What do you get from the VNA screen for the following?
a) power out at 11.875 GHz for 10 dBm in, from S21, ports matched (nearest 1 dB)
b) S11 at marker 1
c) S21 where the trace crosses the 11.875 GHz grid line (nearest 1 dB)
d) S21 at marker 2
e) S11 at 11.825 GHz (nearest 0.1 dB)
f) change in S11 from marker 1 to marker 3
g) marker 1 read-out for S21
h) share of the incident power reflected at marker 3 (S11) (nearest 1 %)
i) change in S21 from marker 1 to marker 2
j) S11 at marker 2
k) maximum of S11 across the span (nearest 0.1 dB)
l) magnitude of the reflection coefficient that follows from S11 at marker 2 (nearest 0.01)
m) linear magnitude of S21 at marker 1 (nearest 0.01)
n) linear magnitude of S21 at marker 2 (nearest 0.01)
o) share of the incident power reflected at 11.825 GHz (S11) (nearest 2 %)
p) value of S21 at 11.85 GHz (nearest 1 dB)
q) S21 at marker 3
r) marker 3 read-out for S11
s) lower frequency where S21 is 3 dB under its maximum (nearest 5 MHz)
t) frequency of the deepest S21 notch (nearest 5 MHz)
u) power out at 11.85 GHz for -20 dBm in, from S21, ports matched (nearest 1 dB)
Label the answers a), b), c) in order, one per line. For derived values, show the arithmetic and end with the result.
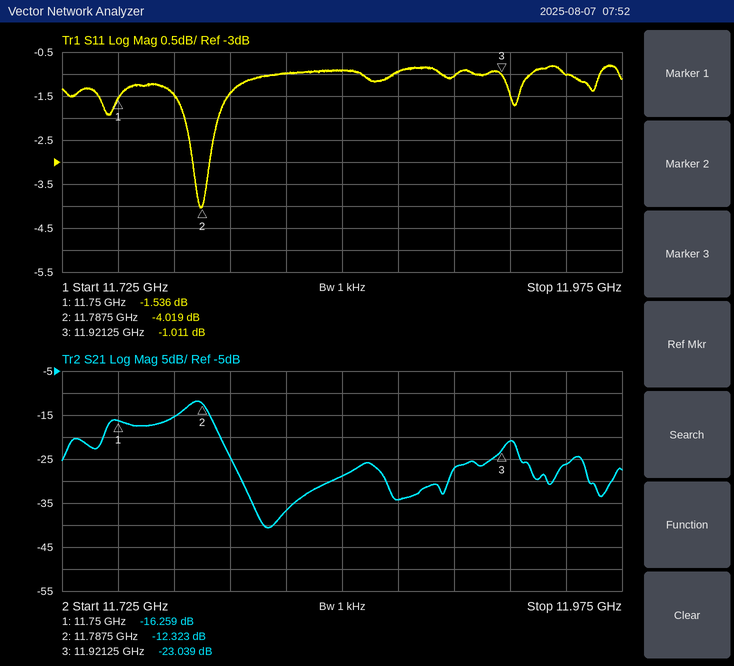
a) 10 dBm + (-34 dB) = -24 dBm
b) -1.536 dB
c) -34 dB
d) -12.323 dB
e) -1.0 dB
f) -1.011 − (-1.536) = 0.525 dB
g) -16.259 dB
h) 10^(-1.011/10) ≈ 79 %
i) -12.323 − (-16.259) = 3.936 dB
j) -4.019 dB
k) -0.8 dB
l) 10^(-4.019/20) ≈ 0.63
m) 10^(-16.259/20) ≈ 0.15
n) 10^(-12.323/20) ≈ 0.24
o) 10^(-1/10) ≈ 79.4 %, so 80 % to the nearest 2 %
p) -29 dB
q) -23.039 dB
r) -1.011 dB
s) 11.775 GHz
t) 11.815 GHz
u) -20 dBm + (-29 dB) = -49 dBm
